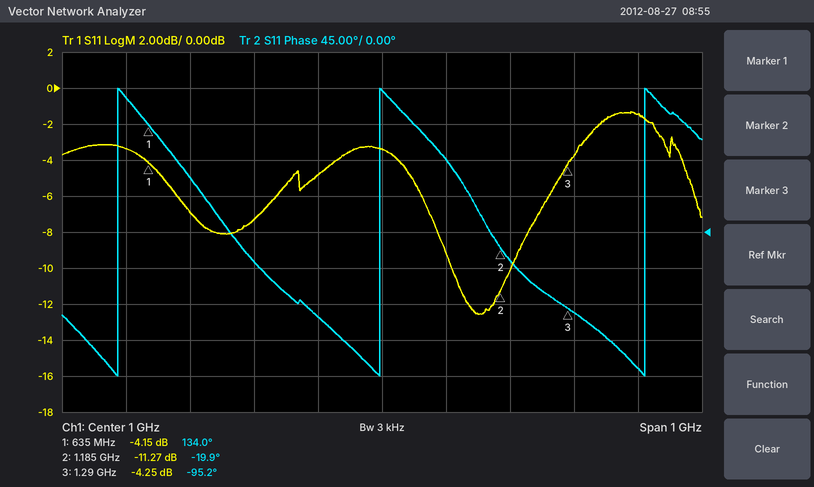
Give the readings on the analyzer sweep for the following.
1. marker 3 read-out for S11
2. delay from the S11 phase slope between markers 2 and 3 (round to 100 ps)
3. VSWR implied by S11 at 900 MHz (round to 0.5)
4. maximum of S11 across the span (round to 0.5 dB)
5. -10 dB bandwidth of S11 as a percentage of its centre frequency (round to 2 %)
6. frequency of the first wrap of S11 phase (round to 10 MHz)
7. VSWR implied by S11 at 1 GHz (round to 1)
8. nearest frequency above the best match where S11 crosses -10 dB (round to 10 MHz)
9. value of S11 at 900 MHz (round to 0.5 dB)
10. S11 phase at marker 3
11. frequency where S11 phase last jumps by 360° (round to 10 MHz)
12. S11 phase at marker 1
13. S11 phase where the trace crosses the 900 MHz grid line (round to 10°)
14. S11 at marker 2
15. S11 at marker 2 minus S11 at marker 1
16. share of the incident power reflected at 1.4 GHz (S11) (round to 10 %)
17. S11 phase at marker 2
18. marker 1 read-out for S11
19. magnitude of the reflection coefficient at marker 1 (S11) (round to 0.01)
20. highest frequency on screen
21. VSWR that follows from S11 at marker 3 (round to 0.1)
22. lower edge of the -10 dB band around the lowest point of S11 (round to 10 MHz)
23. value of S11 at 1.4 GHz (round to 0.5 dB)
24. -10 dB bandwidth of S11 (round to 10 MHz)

-4.25 dB
2.0 ns
3.5
-1.5 dB
8 %
590 MHz
5
1.20 GHz
-5.0 dB
-95.2°
1.41 GHz
134.0°
-110°
-11.27 dB
-7.12 dB
70 %
-19.9°
-4.15 dB
0.62
1.5 GHz
4.2
1.11 GHz
-1.5 dB
90 MHz
